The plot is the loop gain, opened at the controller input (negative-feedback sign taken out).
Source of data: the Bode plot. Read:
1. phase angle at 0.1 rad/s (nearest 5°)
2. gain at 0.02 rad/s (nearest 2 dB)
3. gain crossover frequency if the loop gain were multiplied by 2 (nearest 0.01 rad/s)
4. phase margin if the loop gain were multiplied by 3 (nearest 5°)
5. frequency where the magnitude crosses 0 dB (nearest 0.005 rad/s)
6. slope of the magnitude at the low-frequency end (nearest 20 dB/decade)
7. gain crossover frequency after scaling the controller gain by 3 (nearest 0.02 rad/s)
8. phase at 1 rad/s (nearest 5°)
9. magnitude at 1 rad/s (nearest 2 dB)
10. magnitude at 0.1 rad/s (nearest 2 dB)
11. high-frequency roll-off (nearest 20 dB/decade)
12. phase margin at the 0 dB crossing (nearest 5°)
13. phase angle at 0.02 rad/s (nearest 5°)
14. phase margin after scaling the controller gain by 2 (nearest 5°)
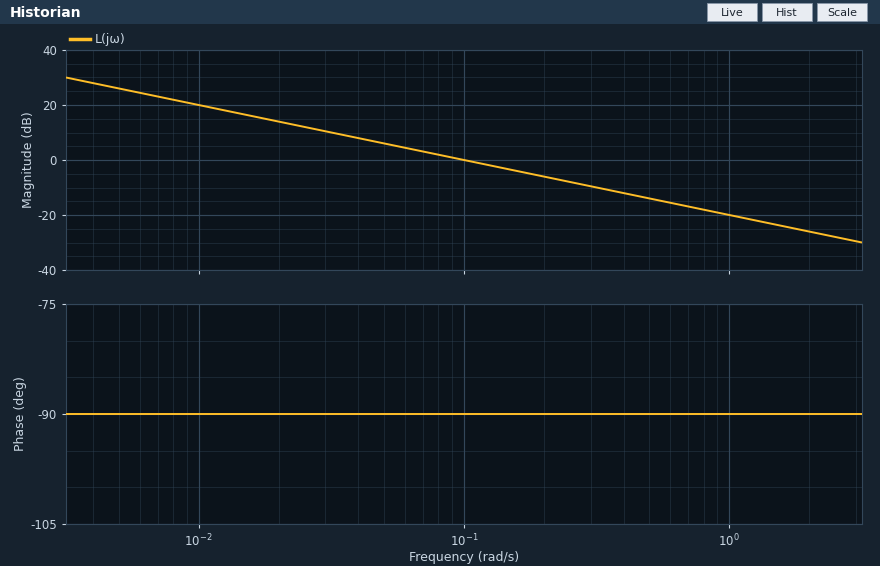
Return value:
-90°
14 dB
0.20 rad/s
90°
0.100 rad/s
-20 dB/decade
0.30 rad/s
-90°
-20 dB
0 dB
-20 dB/decade
90°
-90°
90°
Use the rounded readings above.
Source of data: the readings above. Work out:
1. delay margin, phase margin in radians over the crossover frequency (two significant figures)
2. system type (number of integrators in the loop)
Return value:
16 s
1
